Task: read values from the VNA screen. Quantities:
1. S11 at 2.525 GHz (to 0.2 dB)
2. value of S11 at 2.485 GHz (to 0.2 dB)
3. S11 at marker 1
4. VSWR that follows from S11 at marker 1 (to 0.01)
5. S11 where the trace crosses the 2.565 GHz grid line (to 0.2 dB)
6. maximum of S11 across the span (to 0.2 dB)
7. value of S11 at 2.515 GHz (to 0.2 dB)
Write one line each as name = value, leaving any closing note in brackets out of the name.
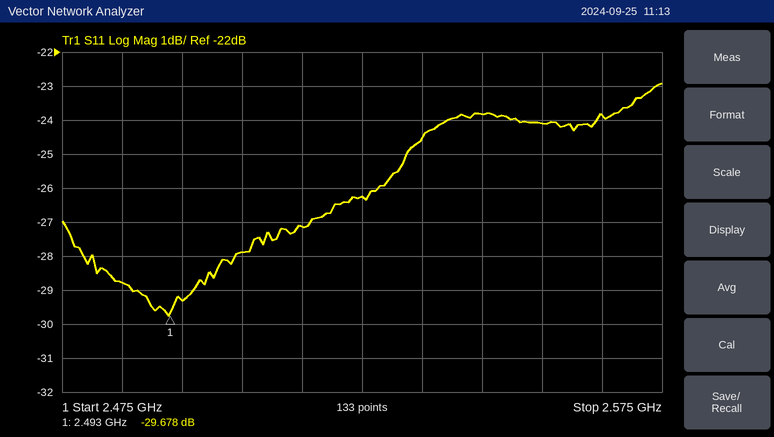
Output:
S11 at 2.525 GHz = -26.2 dB
value of S11 at 2.485 GHz = -28.8 dB
S11 at marker 1 = -29.678 dB
VSWR that follows from S11 at marker 1 = 1.07
S11 where the trace crosses the 2.565 GHz grid line = -23.8 dB
maximum of S11 across the span = -23.0 dB
value of S11 at 2.515 GHz = -27.2 dB
